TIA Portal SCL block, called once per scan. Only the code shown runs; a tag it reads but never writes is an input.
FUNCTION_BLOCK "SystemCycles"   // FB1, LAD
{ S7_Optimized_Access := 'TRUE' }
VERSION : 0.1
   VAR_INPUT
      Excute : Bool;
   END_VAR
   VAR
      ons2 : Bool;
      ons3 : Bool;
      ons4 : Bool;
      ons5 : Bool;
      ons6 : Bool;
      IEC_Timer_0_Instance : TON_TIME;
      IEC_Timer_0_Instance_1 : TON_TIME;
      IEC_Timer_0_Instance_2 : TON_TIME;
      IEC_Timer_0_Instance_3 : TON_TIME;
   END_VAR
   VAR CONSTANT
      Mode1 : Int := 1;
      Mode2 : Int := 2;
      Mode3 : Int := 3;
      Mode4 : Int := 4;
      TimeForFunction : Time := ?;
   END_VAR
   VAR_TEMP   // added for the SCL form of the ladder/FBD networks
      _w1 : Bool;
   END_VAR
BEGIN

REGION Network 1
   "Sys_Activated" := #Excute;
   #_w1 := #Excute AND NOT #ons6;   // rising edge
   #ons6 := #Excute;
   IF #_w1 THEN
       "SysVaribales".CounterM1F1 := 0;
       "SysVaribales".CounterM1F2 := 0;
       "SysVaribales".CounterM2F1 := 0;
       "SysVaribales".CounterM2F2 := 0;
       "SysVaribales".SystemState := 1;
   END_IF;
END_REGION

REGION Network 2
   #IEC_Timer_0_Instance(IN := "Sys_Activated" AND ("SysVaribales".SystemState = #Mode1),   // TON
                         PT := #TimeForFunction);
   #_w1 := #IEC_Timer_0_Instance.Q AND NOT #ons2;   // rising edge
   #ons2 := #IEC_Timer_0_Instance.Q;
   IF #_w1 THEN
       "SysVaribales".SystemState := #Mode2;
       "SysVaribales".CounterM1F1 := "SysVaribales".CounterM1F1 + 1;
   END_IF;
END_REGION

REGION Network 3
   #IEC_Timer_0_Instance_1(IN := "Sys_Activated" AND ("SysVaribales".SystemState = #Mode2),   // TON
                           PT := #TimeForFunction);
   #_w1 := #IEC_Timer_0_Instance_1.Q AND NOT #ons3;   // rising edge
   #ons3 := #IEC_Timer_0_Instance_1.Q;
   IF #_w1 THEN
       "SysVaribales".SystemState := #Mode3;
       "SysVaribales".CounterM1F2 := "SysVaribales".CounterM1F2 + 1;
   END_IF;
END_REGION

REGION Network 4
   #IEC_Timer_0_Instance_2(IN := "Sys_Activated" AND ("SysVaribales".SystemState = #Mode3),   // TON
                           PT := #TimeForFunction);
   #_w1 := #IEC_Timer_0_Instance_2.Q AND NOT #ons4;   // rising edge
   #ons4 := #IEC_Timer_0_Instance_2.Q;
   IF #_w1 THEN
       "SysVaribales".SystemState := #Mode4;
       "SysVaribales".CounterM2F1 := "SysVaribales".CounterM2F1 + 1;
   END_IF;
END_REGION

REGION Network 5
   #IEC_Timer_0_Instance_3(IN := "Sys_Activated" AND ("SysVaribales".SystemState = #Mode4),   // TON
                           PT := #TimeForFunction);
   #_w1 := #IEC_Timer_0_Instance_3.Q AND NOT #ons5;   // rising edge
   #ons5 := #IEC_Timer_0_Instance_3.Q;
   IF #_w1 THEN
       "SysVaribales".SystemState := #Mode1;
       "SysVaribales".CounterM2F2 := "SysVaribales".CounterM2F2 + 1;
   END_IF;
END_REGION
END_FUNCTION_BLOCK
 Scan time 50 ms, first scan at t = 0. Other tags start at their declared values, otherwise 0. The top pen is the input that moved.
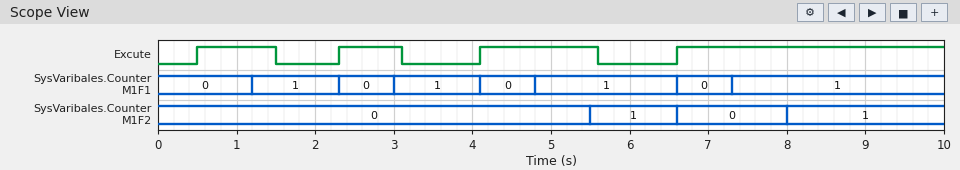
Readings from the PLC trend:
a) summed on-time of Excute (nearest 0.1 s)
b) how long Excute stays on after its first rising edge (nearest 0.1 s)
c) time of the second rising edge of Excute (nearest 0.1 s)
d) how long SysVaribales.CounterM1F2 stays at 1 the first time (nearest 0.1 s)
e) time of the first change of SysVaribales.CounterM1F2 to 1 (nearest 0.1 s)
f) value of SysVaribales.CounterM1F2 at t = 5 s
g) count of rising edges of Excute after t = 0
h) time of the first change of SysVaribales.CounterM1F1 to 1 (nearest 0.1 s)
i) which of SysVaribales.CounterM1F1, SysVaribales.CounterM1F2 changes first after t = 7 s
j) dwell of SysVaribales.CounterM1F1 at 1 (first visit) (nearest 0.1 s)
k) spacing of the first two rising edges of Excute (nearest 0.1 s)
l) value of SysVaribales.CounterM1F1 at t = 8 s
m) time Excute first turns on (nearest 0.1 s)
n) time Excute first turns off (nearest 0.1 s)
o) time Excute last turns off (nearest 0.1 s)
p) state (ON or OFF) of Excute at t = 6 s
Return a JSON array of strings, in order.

["6.7 s", "1.0 s", "2.3 s", "1.1 s", "5.5 s", "0", "4", "1.2 s", "SysVaribales.CounterM1F1", "1.1 s", "1.8 s", "1", "0.5 s", "1.5 s", "5.6 s", "OFF"]
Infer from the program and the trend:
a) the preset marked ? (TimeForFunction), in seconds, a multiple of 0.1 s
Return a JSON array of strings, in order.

["0.7 s"]
